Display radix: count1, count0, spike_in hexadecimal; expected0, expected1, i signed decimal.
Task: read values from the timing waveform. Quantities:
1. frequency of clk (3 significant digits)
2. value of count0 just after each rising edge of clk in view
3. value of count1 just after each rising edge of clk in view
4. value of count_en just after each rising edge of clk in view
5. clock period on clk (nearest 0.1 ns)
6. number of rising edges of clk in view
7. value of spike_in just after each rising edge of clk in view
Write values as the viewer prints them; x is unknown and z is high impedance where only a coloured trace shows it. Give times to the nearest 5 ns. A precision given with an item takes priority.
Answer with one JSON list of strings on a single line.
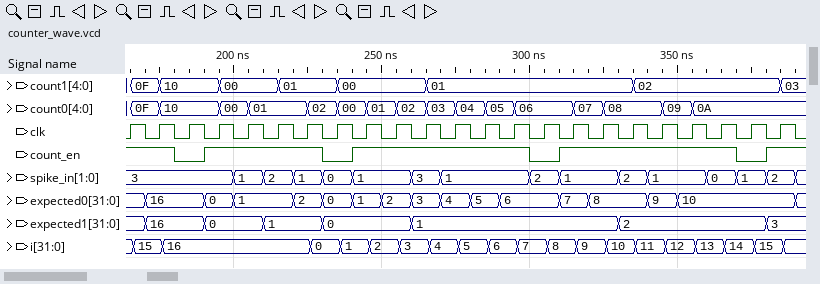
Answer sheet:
["100 MHz", "0F, 10, 10, 00, 01, 01, 02, 00, 01, 02, 03, 04, 05, 06, 06, 07, 08, 08, 09, 0A, 0A, 0A, 0A", "0F, 10, 10, 00, 00, 01, 01, 00, 00, 00, 01, 01, 01, 01, 01, 01, 01, 02, 02, 02, 02, 02, 03", "1 1 0 1 1 1 1 0 1 1 1 1 1 1 0 1 1 1 1 1 1 0 1", "10 ns", "23", "3, 3, 3, 3, 1, 2, 1, 0, 1, 1, 3, 1, 1, 1, 2, 1, 1, 2, 1, 1, 0, 1, 2"]
